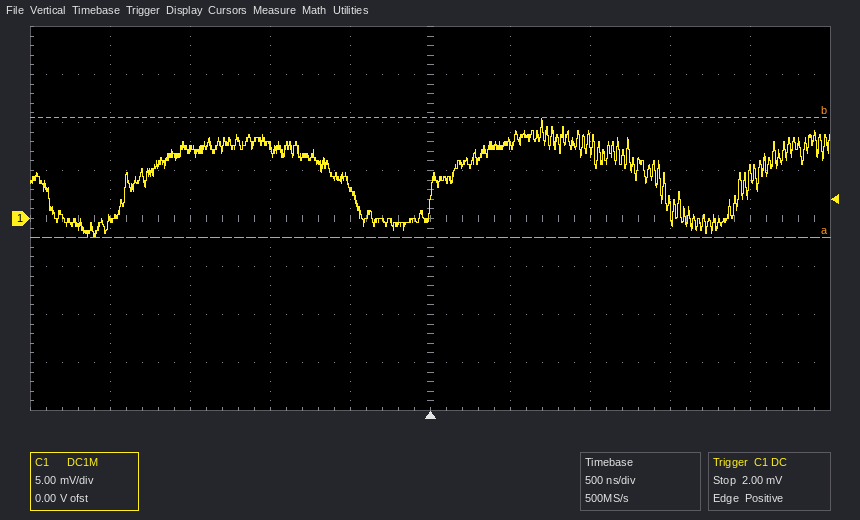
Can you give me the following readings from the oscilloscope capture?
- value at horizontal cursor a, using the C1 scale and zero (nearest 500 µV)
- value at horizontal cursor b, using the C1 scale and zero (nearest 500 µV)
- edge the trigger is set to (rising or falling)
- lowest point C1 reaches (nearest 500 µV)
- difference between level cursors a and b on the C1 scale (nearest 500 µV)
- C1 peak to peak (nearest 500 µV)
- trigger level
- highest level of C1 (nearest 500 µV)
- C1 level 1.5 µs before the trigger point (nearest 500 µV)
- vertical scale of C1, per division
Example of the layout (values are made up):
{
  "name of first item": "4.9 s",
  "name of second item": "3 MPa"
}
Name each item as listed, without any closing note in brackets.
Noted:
{
  "value at horizontal cursor a, using the C1 scale and zero": "-2.0 mV",
  "value at horizontal cursor b, using the C1 scale and zero": "10.5 mV",
  "edge the trigger is set to": "rising",
  "lowest point C1 reaches": "-2.0 mV",
  "difference between level cursors a and b on the C1 scale": "12.5 mV",
  "C1 peak to peak": "12.5 mV",
  "trigger level": "2.00 mV",
  "highest level of C1": "10.5 mV",
  "C1 level 1.5 µs before the trigger point": "7.0 mV",
  "vertical scale of C1, per division": "5 mV"
}
